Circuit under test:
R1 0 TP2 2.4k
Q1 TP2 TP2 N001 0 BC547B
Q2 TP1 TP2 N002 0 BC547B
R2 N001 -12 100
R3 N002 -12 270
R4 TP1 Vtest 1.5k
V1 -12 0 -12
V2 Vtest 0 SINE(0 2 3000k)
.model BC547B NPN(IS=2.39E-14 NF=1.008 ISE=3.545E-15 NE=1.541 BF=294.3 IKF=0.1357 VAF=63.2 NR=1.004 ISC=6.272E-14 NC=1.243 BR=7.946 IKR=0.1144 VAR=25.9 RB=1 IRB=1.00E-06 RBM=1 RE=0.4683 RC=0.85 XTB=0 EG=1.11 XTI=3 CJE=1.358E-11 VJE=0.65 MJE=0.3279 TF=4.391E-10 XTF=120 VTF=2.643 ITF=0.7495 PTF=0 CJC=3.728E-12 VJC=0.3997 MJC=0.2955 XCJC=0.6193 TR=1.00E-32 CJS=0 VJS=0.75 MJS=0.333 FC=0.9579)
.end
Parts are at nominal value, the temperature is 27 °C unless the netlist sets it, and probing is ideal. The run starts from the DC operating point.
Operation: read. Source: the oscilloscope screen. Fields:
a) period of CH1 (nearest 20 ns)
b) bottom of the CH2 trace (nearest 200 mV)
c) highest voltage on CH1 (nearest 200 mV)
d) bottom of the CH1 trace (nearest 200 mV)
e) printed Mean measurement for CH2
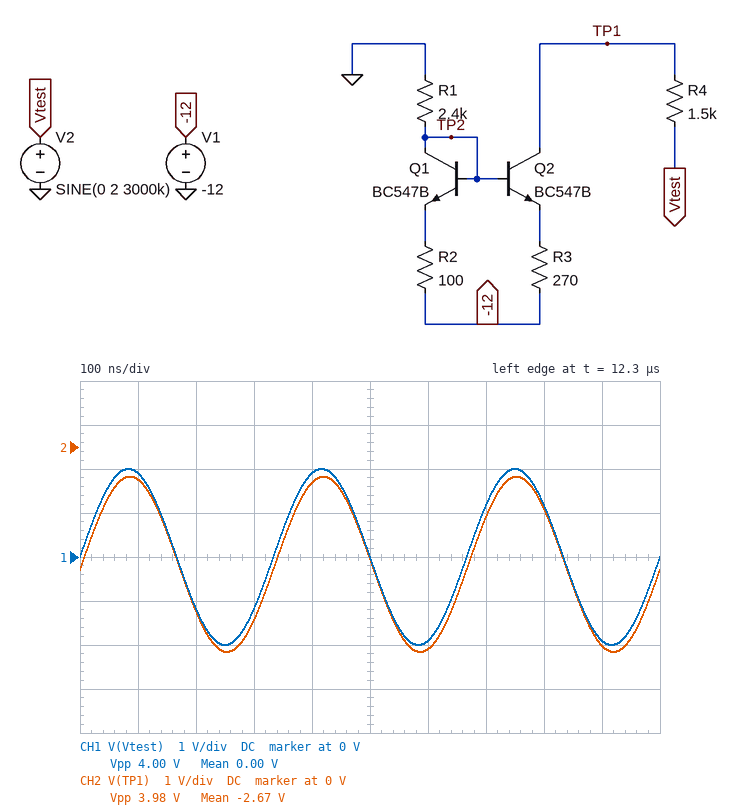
340 ns
-4.6 V
2.0 V
-2.0 V
-2.67 V
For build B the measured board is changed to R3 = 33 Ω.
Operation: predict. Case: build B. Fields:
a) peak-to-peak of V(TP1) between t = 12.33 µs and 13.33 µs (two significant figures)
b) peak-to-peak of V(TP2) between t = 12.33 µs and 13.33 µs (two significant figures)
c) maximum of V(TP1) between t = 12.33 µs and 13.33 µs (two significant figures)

81 mV
63 mV
-12 V
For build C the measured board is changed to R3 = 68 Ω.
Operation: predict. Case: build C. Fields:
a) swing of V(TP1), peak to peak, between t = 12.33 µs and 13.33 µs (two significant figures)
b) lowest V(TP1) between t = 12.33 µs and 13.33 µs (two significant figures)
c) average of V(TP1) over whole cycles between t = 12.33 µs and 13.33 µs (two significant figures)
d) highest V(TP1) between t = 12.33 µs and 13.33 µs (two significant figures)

3.7 V
-11 V
-9.7 V
-7.7 V
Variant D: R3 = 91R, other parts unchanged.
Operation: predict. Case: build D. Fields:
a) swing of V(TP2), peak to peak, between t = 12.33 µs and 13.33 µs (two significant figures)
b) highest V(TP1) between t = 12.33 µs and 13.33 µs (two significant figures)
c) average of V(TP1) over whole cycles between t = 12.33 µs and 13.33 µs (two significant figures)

15 mV
-5.4 V
-7.4 V
